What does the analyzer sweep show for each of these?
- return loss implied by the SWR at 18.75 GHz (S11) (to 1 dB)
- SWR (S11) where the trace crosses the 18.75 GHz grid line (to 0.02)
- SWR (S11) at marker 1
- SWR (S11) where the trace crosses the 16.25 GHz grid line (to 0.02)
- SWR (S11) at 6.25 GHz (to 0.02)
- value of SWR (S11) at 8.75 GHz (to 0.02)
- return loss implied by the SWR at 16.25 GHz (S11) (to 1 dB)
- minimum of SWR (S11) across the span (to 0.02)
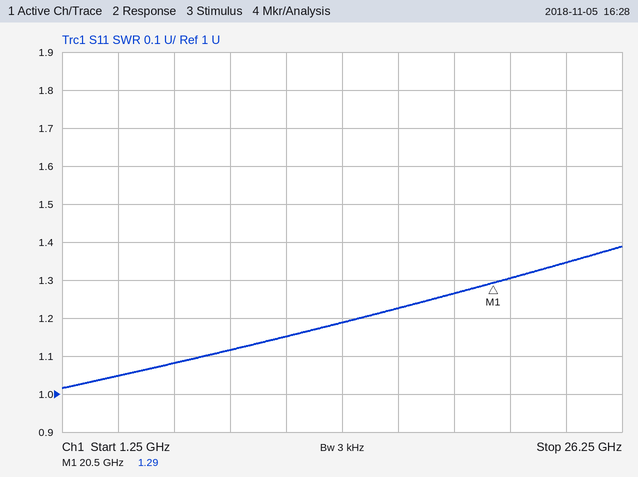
19 dB
1.26
1.29
1.22
1.08
1.12
20 dB
1.02
